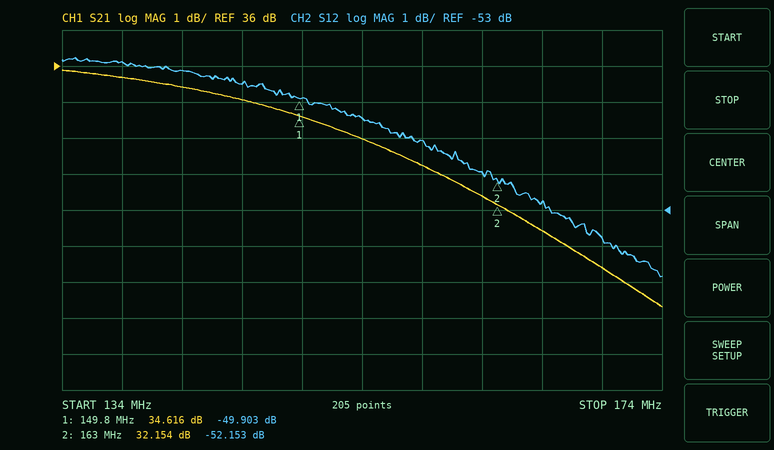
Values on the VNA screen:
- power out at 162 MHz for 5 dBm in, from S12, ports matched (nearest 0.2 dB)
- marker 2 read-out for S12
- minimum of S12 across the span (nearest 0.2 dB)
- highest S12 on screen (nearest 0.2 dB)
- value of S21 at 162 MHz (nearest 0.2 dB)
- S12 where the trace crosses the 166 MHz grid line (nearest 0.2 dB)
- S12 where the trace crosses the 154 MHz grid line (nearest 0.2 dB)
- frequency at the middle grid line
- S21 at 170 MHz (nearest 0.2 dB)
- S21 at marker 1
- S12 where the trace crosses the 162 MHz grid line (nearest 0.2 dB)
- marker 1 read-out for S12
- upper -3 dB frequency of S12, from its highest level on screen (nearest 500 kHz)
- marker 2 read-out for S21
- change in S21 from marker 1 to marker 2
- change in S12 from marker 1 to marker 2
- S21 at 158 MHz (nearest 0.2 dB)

-47.0 dBm
-52.153 dB
-54.8 dB
-48.8 dB
32.4 dB
-52.8 dB
-50.4 dB
154 MHz
30.4 dB
34.616 dB
-52.0 dB
-49.903 dB
161.0 MHz
32.154 dB
-2.462 dB
-2.250 dB
33.2 dB
